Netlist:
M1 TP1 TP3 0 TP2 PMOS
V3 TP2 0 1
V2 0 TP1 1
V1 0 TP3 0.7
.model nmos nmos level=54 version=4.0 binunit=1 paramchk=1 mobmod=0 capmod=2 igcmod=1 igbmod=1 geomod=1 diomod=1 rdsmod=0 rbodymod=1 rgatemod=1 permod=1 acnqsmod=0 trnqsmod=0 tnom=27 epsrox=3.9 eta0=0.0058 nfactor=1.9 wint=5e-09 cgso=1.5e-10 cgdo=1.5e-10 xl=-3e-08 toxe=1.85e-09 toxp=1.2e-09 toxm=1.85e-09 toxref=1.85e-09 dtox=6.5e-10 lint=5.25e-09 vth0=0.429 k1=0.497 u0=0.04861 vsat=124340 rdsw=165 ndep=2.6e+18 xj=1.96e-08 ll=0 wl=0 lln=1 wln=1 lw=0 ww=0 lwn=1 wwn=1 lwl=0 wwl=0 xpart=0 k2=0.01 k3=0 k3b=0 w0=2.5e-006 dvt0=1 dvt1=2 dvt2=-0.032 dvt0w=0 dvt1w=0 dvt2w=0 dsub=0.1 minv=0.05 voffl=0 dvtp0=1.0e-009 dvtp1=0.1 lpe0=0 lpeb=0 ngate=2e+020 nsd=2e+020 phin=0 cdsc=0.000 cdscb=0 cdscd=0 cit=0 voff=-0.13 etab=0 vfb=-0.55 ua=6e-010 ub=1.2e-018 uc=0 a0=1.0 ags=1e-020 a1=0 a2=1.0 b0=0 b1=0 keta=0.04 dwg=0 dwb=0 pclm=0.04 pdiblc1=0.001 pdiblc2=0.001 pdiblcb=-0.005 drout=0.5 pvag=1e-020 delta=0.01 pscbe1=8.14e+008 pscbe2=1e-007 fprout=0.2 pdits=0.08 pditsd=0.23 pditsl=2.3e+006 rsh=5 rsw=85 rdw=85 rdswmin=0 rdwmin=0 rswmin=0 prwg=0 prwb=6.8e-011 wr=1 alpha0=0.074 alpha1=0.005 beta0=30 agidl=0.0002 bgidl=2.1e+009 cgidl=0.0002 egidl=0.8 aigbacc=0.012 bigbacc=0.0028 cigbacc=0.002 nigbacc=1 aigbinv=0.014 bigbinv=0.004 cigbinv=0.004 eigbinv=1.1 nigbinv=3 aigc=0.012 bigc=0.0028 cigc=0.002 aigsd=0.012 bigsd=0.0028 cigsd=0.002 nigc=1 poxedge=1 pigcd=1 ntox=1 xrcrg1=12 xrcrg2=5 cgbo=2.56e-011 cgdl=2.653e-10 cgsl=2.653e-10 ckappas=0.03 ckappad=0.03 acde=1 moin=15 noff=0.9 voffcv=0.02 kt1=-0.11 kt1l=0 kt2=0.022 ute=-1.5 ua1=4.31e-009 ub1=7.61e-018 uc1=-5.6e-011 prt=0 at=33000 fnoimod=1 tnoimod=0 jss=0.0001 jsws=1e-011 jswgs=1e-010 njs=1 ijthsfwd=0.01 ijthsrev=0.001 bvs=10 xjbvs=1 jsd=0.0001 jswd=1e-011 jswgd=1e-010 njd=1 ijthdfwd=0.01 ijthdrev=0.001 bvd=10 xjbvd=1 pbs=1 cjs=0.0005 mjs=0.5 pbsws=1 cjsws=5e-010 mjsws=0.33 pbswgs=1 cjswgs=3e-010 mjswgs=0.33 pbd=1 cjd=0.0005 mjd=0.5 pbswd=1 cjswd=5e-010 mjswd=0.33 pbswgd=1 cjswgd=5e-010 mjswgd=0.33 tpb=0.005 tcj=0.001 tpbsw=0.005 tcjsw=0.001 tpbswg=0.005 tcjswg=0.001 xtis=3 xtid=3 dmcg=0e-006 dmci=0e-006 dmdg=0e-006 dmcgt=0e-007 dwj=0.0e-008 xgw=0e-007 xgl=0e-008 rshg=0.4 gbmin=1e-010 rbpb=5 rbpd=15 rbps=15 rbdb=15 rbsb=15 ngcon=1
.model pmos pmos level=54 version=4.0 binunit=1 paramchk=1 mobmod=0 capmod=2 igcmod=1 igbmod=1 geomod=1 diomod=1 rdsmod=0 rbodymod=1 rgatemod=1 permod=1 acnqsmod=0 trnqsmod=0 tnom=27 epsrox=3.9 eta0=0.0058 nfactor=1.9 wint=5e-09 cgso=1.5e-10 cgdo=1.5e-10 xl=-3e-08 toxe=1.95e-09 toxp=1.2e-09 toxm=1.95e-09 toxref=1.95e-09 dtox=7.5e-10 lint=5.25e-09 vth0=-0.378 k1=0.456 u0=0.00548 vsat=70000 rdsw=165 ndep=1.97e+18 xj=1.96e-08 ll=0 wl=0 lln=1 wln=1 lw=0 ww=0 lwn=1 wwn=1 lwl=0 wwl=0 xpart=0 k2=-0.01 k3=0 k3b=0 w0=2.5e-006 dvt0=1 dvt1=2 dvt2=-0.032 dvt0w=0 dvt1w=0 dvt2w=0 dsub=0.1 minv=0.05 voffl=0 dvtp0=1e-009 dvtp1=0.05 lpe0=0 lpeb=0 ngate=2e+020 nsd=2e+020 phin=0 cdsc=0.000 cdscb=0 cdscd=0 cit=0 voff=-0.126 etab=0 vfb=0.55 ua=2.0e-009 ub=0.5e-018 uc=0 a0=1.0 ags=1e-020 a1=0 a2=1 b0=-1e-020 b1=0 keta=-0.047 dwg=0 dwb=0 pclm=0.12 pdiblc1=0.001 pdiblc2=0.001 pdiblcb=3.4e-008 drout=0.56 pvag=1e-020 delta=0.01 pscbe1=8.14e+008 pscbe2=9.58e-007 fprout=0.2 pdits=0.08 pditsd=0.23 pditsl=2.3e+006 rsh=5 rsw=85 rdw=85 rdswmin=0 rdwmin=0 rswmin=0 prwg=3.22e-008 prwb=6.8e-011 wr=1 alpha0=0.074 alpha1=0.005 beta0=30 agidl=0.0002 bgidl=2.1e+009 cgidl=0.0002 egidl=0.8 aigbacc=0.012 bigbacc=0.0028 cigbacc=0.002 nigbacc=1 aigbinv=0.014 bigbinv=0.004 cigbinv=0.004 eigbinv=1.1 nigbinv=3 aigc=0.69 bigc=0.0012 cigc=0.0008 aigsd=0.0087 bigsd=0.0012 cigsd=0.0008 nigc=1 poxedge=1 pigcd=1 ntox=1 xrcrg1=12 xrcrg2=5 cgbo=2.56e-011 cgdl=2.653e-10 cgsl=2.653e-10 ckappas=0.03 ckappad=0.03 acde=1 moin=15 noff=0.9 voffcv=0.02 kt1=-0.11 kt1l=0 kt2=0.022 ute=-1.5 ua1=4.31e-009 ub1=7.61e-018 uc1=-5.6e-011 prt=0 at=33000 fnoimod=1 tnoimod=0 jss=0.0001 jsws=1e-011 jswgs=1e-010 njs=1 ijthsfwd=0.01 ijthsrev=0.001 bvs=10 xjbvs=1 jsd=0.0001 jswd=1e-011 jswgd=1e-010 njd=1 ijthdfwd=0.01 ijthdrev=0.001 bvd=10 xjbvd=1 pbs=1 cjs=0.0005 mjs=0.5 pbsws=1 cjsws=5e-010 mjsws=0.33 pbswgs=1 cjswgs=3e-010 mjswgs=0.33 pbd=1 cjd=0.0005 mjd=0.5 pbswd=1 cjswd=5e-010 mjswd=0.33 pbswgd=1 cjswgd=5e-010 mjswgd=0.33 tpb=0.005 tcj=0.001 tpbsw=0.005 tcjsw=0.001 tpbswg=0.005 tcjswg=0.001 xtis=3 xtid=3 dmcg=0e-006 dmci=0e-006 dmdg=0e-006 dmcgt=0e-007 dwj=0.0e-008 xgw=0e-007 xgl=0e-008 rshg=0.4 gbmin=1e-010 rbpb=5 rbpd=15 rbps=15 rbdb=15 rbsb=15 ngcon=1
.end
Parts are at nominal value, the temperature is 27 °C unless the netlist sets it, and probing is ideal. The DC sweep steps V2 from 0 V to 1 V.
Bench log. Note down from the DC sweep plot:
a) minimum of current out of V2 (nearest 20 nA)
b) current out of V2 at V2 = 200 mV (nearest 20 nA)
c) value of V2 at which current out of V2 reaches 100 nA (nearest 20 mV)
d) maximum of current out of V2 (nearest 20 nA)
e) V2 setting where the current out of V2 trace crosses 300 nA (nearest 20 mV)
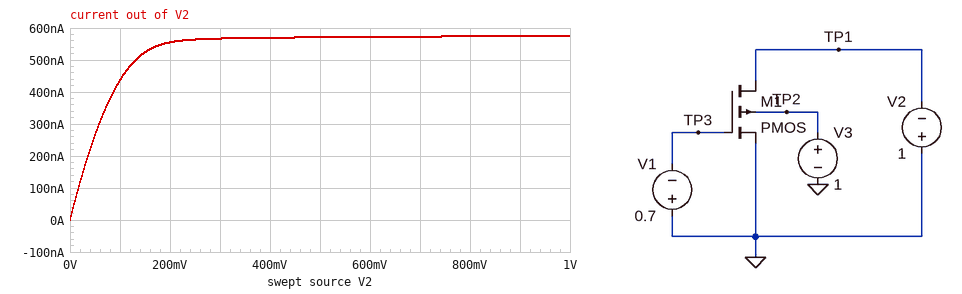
0 A
560 nA
20 mV
580 nA
60 mV
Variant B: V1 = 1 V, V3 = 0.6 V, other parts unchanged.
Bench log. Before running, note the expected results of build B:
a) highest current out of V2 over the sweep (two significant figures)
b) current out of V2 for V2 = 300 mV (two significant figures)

5.7 µA
4.7 µA
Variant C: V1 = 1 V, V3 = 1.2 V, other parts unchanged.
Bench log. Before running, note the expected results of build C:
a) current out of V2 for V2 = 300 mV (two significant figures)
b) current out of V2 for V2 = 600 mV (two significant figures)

3.3 µA
3.7 µA
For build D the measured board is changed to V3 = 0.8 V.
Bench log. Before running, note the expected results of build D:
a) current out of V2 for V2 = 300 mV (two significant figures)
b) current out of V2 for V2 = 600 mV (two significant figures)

810 nA
820 nA
